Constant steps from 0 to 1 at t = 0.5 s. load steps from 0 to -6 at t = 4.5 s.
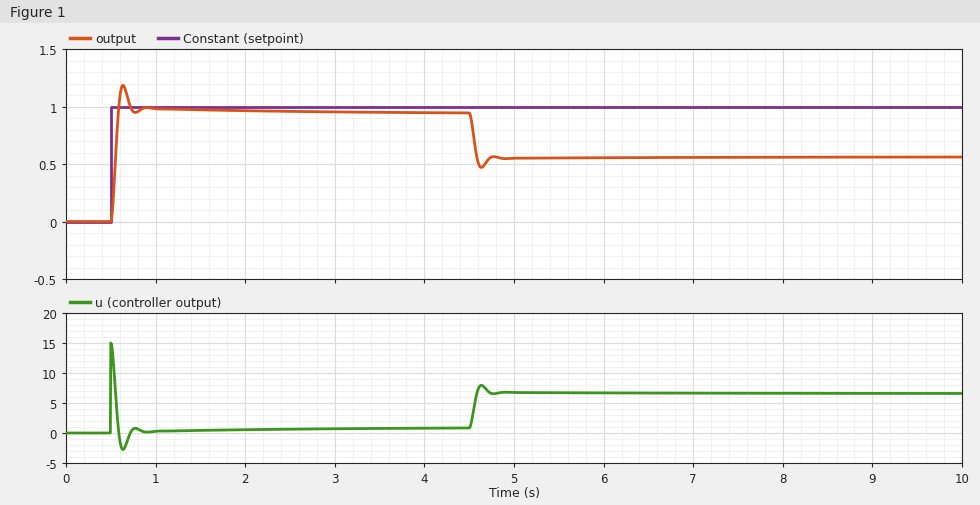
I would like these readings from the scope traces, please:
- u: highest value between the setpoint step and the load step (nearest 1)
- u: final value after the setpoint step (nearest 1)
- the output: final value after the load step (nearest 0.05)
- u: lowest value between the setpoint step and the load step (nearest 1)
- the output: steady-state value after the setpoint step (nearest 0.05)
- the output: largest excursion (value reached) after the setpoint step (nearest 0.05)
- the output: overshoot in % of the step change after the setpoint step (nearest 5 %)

15
1
0.55
-3
0.95
1.20
25 %
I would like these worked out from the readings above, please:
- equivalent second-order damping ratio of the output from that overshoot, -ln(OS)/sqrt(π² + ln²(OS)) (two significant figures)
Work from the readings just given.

0.40
